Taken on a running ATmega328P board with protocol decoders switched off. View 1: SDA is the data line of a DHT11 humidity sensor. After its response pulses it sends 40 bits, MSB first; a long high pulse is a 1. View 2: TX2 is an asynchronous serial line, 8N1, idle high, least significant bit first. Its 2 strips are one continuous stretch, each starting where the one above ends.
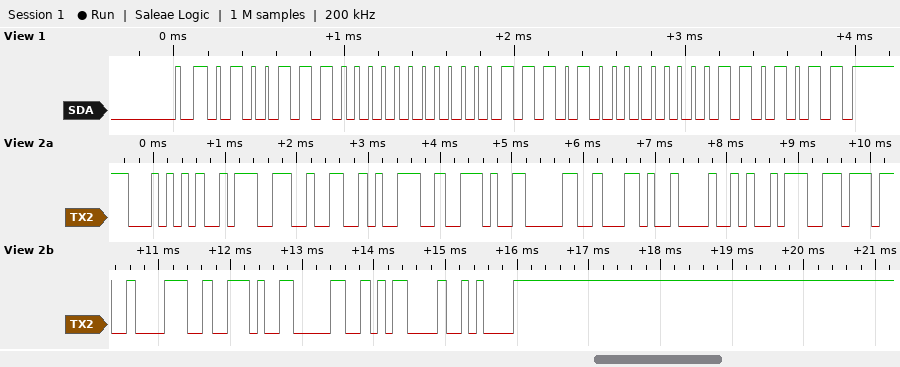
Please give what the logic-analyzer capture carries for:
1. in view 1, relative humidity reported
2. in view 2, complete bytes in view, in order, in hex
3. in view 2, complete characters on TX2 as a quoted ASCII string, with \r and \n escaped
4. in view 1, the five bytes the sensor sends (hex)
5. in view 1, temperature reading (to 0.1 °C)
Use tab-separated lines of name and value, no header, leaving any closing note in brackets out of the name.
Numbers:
in view 1, relative humidity reported	78 %
in view 2, complete bytes in view, in order, in hex	0x54 0x3A 0x32 0x39 0x2E 0x30 0x2C 0x48 0x3A 0x37 0x38 0x2E 0x30 0x0D 0x0A
in view 2, complete characters on TX2 as a quoted ASCII string, with \r and \n escaped	"T:29.0,H:78.0\r\n"
in view 1, the five bytes the sensor sends	4E 00 1D 00 6B
in view 1, temperature reading	29.0 °C
